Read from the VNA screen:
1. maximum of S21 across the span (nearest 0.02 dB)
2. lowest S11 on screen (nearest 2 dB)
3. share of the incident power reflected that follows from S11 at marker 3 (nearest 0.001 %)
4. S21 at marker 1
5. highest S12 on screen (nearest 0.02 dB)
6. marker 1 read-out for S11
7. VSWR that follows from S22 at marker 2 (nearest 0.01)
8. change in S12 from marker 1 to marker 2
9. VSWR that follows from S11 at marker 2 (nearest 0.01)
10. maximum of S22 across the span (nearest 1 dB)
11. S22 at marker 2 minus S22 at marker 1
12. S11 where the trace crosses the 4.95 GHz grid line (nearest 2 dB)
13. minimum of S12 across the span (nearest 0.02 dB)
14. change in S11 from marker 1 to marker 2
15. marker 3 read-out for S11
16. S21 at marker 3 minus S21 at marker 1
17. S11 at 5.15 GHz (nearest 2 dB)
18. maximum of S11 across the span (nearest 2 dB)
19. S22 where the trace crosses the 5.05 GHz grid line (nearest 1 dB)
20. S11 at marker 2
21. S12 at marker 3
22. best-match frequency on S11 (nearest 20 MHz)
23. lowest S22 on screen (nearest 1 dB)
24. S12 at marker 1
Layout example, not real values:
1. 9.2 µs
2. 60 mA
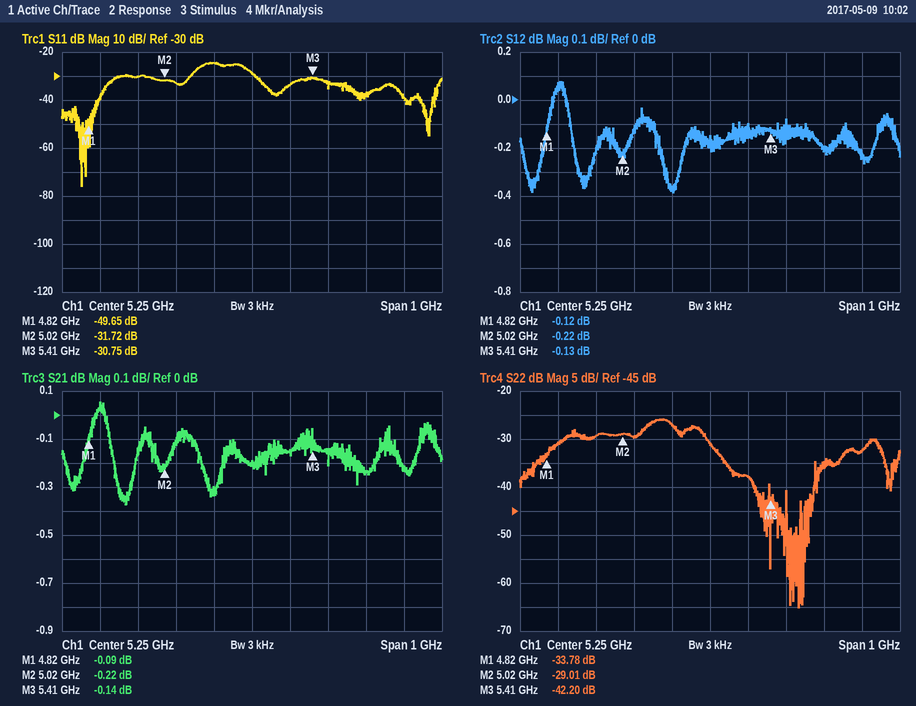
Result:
1. 0.06 dB
2. -76 dB
3. 0.084 %
4. -0.09 dB
5. 0.08 dB
6. -49.65 dB
7. 1.07
8. -0.10 dB
9. 1.05
10. -26 dB
11. 4.77 dB
12. -30 dB
13. -0.38 dB
14. 17.93 dB
15. -30.75 dB
16. -0.05 dB
17. -24 dB
18. -24 dB
19. -30 dB
20. -31.72 dB
21. -0.13 dB
22. 4.80 GHz
23. -65 dB
24. -0.12 dB
